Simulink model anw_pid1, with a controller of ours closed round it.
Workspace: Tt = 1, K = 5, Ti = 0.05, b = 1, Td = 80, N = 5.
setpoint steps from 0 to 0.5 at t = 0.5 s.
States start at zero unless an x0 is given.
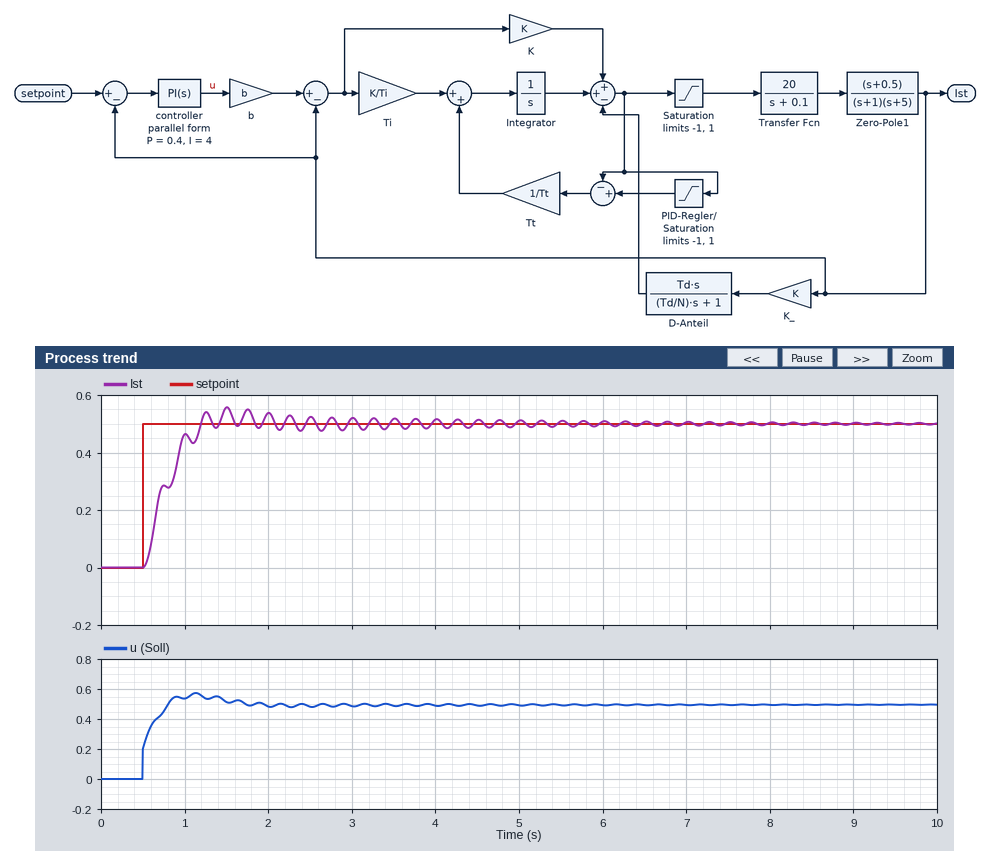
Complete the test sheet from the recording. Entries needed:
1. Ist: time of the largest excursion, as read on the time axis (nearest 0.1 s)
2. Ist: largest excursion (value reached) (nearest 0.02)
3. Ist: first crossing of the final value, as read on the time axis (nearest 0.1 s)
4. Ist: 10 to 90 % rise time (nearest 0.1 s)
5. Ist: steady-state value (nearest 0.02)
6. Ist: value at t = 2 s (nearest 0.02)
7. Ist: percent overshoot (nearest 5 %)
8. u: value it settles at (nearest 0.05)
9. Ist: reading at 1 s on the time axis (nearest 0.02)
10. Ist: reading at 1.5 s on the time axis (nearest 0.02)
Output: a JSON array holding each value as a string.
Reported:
["1.5 s", "0.56", "1.2 s", "0.4 s", "0.50", "0.54", "10 %", "0.50", "0.46", "0.56"]
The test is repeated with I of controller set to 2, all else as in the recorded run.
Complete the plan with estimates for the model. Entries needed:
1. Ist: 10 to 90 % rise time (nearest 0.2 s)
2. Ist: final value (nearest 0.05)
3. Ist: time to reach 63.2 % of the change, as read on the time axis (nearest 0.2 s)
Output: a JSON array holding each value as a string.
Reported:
["0.8 s", "0.50", "1.0 s"]
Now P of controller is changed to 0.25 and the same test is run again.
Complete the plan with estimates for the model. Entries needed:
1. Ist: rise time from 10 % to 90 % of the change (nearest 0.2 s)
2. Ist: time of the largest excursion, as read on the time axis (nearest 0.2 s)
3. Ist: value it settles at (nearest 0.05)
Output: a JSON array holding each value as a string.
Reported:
["0.6 s", "1.4 s", "0.50"]
